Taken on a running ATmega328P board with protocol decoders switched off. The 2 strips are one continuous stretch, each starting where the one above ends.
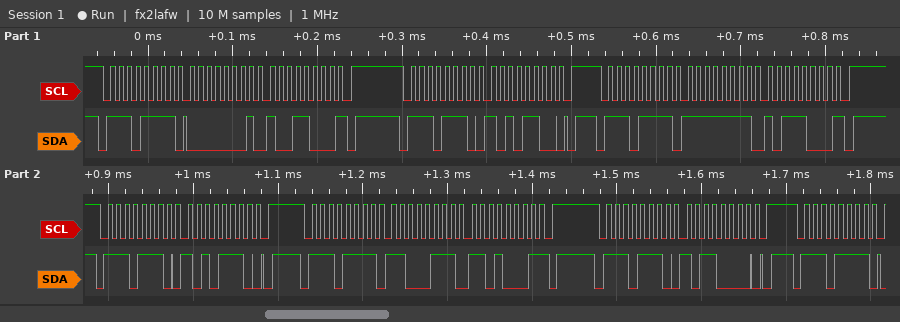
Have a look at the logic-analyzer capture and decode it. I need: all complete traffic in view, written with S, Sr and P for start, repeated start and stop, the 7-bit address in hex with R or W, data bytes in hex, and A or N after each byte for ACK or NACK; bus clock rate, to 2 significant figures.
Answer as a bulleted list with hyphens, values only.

- S 77R A 01 A 98 N P S 77W A AC A P S 77R A FF A B8 N P S 77W A AE A P S 77R A C7 A D1 N P S 77W A B0 A P S 77R A
- 100 kHz
